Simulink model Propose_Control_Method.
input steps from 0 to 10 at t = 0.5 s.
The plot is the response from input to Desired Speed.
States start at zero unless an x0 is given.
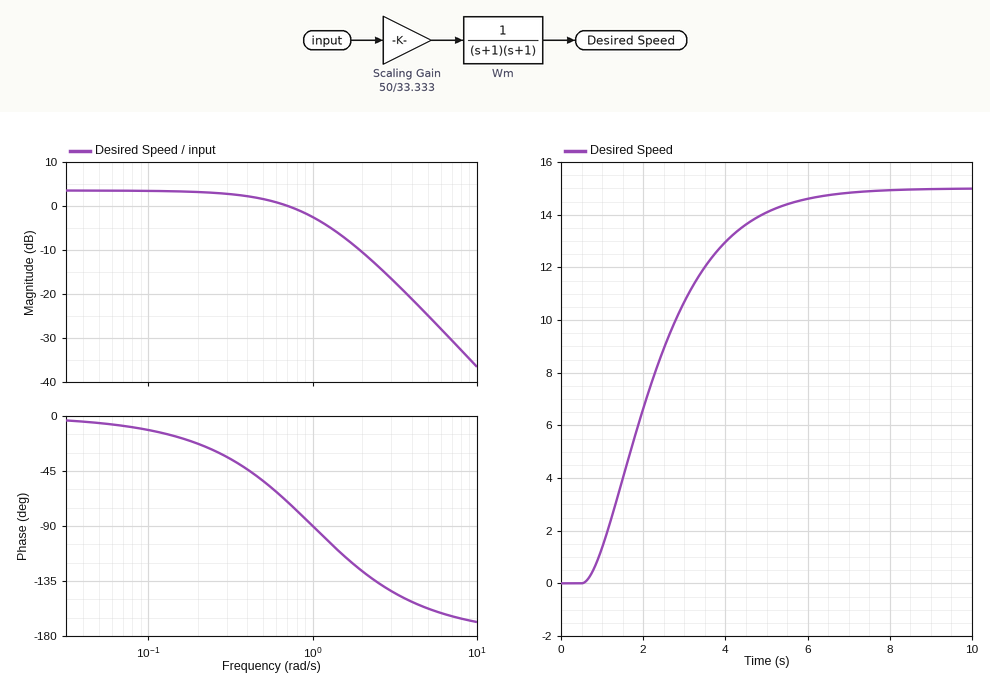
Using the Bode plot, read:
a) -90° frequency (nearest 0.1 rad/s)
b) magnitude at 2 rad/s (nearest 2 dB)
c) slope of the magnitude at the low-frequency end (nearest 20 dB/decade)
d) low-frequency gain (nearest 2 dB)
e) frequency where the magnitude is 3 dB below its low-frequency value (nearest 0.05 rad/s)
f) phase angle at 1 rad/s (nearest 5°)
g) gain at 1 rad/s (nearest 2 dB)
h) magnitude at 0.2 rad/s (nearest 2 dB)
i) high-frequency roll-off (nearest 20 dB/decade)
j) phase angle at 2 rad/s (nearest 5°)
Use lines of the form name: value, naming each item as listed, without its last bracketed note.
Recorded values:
-90° frequency: 1.0 rad/s
magnitude at 2 rad/s: -10 dB
slope of the magnitude at the low-frequency end: 0 dB/decade
low-frequency gain: 4 dB
frequency where the magnitude is 3 dB below its low-frequency value: 0.65 rad/s
phase angle at 1 rad/s: -90°
gain at 1 rad/s: -2 dB
magnitude at 0.2 rad/s: 4 dB
high-frequency roll-off: -40 dB/decade
phase angle at 2 rad/s: -125°
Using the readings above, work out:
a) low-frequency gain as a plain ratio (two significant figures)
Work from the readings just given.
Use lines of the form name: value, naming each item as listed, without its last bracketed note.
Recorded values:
low-frequency gain as a plain ratio: 1.6
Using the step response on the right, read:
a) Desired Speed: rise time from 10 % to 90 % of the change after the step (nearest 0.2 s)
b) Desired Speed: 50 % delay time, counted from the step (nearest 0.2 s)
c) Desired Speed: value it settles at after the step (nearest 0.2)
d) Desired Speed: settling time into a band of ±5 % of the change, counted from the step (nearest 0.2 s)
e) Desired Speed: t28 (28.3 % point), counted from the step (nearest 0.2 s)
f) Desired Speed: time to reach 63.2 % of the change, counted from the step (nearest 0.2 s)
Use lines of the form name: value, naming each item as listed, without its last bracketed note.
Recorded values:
Desired Speed: rise time from 10 % to 90 % of the change after the step: 3.4 s
Desired Speed: 50 % delay time, counted from the step: 1.6 s
Desired Speed: value it settles at after the step: 15.0
Desired Speed: settling time into a band of ±5 % of the change, counted from the step: 4.8 s
Desired Speed: t28 (28.3 % point), counted from the step: 1.0 s
Desired Speed: time to reach 63.2 % of the change, counted from the step: 2.2 s
